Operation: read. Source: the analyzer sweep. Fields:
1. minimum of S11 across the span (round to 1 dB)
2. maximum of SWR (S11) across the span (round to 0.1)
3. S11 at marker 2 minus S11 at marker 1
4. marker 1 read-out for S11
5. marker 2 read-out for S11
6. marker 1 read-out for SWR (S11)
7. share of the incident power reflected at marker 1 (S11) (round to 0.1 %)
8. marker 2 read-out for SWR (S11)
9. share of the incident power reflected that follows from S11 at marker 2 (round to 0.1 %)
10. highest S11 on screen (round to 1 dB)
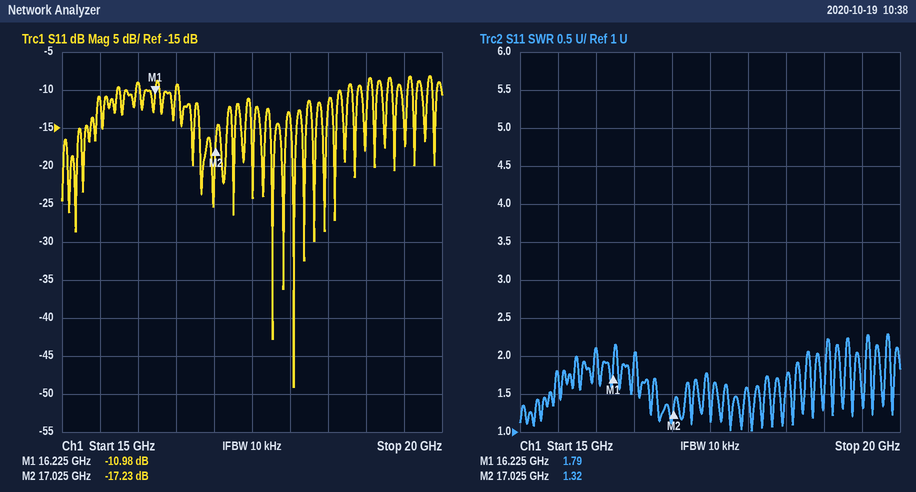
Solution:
-49 dB
2.3
-6.25 dB
-10.98 dB
-17.23 dB
1.79
8.0 %
1.32
1.9 %
-8 dB
